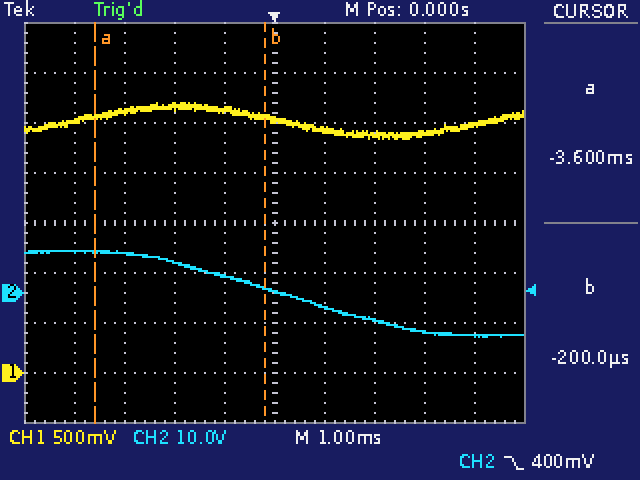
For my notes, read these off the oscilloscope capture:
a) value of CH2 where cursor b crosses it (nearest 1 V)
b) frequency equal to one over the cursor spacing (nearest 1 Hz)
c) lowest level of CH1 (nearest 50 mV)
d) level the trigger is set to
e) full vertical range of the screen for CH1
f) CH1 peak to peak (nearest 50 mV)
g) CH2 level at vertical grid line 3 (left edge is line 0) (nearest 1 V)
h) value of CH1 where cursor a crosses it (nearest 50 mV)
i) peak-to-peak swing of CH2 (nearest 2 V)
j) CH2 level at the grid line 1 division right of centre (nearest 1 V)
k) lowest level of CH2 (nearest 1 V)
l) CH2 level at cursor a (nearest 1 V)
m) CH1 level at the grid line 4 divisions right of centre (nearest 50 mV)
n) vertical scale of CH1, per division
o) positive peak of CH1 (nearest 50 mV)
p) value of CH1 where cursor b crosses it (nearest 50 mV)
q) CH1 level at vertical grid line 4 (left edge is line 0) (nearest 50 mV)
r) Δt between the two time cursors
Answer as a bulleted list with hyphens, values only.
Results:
- 1 V
- 294 Hz
- 2.35 V
- 400 mV
- 4 V
- 350 mV
- 6 V
- 2.55 V
- 18 V
- -3 V
- -9 V
- 8 V
- 2.50 V
- 500 mV
- 2.70 V
- 2.55 V
- 2.65 V
- 3.4 ms
